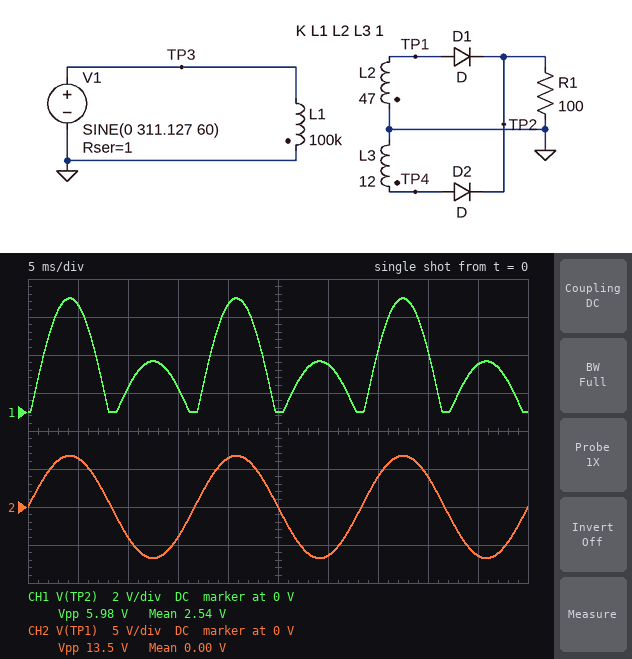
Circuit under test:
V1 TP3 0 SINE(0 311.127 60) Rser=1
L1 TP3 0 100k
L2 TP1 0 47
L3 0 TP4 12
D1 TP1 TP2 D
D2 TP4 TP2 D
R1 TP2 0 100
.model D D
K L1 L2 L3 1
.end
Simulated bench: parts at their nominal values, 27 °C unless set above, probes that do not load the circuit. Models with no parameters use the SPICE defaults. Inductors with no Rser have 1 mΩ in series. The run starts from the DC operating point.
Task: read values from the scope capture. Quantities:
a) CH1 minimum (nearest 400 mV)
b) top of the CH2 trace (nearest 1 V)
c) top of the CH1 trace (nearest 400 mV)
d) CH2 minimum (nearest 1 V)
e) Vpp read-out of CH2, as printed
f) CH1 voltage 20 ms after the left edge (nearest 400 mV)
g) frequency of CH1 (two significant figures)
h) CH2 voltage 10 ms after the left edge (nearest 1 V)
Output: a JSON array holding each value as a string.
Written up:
["0 V", "7 V", "6.0 V", "-7 V", "13.5 V", "5.6 V", "60 Hz", "-4 V"]
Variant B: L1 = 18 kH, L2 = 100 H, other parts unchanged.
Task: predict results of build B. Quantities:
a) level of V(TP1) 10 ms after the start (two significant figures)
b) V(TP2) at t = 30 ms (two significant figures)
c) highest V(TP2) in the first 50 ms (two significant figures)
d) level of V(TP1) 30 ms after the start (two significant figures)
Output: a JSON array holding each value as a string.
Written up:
["-14 V", "6.9 V", "22 V", "-22 V"]
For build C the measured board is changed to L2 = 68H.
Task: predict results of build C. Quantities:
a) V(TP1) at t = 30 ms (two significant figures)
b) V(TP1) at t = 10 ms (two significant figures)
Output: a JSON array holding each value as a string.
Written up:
["-7.7 V", "-4.8 V"]
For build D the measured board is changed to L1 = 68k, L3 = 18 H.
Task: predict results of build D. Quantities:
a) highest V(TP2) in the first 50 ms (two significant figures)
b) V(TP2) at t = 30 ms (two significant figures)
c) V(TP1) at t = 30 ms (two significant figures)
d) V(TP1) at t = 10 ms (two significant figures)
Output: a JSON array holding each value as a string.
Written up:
["7.4 V", "4.1 V", "-7.8 V", "-4.8 V"]
